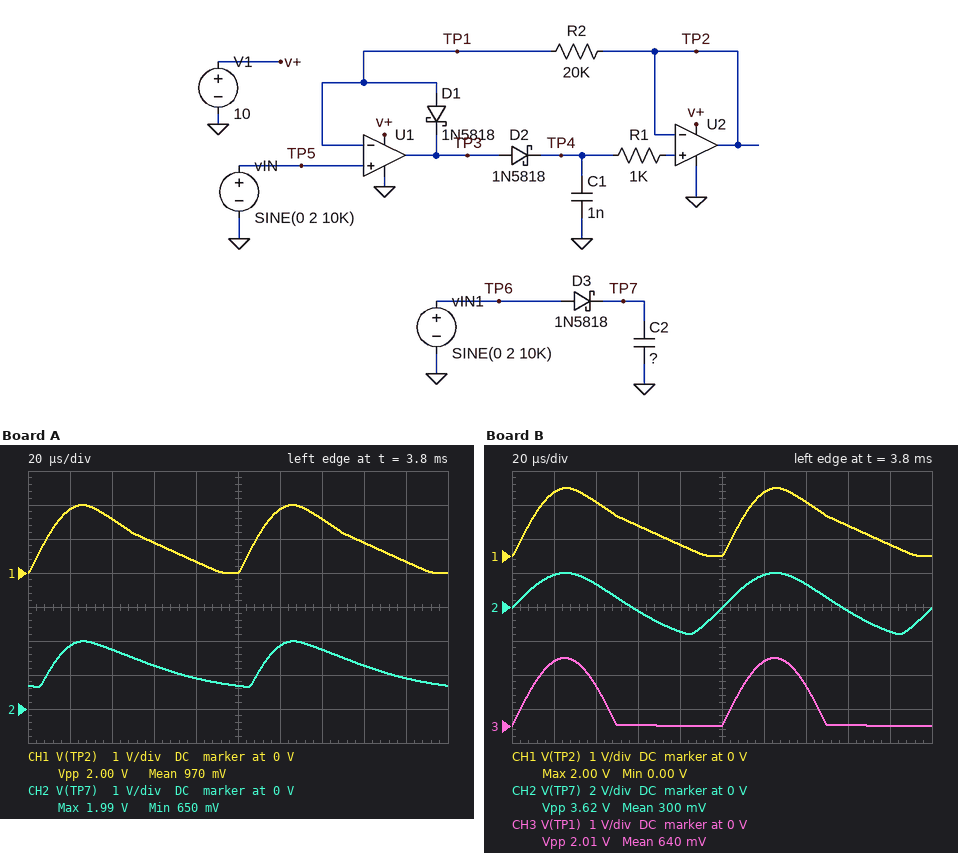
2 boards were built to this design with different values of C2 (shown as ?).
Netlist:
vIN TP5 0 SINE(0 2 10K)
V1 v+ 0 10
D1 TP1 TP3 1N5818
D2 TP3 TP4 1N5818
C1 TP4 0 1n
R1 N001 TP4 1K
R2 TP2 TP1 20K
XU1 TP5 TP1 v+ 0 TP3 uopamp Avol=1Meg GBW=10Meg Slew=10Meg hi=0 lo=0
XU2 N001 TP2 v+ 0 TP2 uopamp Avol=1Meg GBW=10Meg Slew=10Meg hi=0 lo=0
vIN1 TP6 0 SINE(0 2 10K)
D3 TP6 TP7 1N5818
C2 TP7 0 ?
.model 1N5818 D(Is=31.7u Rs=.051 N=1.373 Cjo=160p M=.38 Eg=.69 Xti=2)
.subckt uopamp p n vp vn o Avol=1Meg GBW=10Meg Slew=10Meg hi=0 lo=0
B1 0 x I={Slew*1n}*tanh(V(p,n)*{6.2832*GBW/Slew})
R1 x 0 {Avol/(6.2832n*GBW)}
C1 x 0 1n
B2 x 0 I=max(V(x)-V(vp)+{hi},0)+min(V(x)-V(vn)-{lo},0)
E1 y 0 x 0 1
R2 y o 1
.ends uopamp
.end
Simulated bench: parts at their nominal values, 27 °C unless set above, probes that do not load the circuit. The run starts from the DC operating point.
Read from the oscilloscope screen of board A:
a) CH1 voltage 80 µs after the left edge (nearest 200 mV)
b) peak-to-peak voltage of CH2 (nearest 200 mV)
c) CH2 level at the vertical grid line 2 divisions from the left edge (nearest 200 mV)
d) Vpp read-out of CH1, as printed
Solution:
400 mV
1.4 V
1.8 V
2.00 V
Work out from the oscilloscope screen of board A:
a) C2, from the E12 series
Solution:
1.8 nF
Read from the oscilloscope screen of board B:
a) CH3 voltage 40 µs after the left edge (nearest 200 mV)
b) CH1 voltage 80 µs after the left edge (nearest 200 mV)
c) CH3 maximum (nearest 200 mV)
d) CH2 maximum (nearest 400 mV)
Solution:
1.2 V
400 mV
2.0 V
2.0 V
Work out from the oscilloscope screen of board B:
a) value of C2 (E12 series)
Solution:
470 pF
